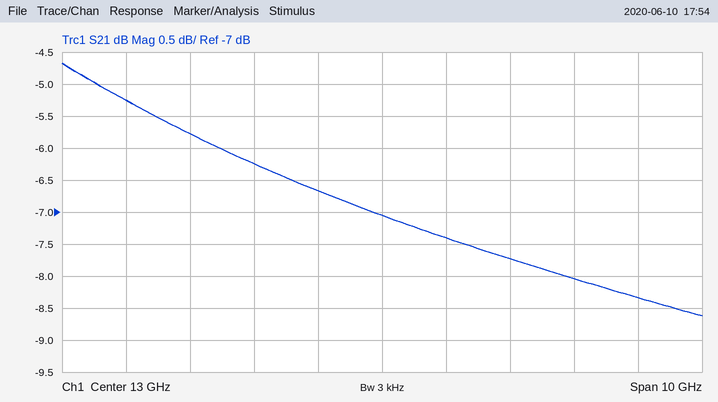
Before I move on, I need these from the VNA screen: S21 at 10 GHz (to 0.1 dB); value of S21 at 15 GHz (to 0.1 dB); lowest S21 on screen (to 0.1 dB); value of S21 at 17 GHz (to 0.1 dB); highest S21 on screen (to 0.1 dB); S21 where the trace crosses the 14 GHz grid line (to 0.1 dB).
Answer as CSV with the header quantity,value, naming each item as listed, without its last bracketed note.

quantity,value
S21 at 10 GHz,-5.8 dB
value of S21 at 15 GHz,-7.7 dB
lowest S21 on screen,-8.6 dB
value of S21 at 17 GHz,-8.3 dB
highest S21 on screen,-4.7 dB
S21 where the trace crosses the 14 GHz grid line,-7.4 dB
